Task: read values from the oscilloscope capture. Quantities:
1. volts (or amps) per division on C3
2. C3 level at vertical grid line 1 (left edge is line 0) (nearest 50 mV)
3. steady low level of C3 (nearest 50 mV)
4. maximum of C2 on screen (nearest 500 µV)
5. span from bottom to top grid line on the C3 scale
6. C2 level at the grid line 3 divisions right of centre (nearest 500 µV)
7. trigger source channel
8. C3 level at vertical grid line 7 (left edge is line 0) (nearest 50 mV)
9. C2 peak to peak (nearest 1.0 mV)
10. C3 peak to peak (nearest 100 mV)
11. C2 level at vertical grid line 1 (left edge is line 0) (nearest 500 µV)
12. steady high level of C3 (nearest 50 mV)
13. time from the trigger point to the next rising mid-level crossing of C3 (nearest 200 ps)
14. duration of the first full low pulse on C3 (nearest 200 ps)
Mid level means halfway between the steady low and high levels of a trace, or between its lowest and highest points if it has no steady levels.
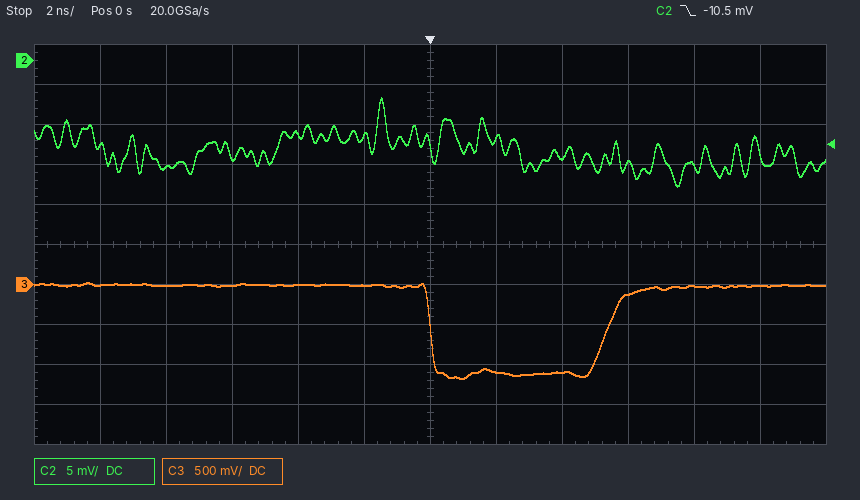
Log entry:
500 mV
0 mV
-1.10 V
-4.5 mV
5 V
-13.0 mV
C2
-1.10 V
11.0 mV
1.20 V
-10.5 mV
0 mV
5.4 ns
5.4 ns
